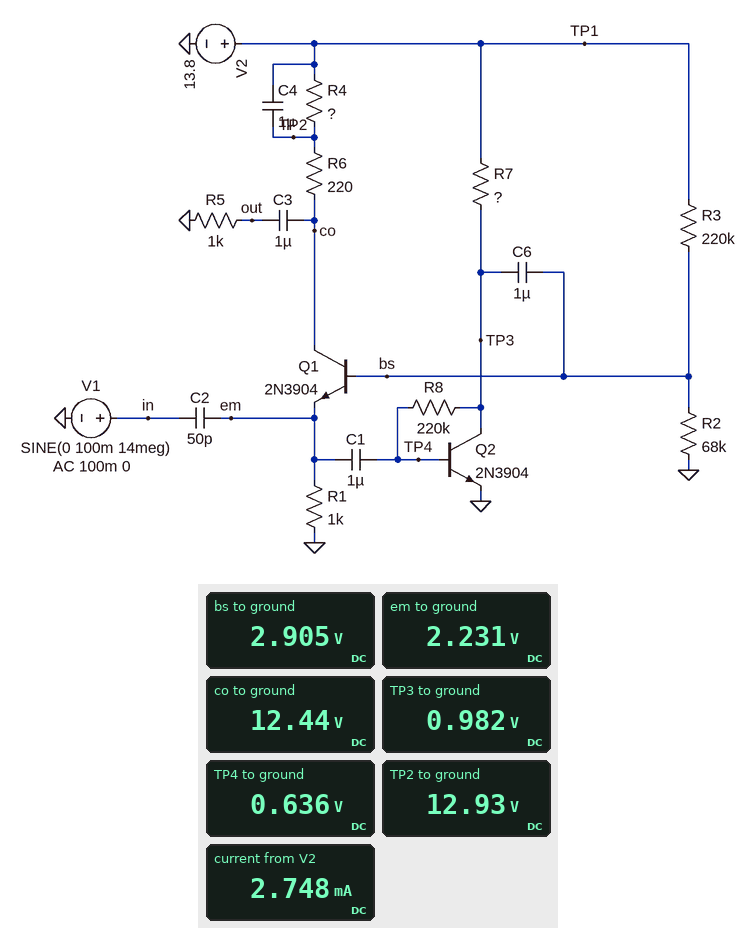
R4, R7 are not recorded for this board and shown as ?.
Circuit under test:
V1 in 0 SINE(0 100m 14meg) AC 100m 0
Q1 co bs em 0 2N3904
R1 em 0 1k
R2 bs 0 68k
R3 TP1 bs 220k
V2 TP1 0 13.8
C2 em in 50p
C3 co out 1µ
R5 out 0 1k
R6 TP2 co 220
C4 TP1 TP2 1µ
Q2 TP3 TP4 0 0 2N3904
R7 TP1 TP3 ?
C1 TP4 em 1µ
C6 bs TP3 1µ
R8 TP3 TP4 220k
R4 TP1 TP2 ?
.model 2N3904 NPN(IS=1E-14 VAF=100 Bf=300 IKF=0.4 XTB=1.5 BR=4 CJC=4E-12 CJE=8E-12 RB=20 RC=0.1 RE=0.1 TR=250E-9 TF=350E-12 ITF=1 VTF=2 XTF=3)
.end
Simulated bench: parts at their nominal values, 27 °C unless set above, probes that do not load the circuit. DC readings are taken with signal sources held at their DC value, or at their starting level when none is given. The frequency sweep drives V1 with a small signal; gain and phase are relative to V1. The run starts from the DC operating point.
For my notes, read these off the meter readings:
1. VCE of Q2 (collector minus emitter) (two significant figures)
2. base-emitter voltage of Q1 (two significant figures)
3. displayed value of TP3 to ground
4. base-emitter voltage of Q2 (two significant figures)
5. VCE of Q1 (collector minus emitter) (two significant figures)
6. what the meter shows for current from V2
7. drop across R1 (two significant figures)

980 mV
670 mV
0.982 V
640 mV
10 V
2.748 mA
2.2 V
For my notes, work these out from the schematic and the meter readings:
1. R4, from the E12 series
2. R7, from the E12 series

390 Ω
27 kΩ
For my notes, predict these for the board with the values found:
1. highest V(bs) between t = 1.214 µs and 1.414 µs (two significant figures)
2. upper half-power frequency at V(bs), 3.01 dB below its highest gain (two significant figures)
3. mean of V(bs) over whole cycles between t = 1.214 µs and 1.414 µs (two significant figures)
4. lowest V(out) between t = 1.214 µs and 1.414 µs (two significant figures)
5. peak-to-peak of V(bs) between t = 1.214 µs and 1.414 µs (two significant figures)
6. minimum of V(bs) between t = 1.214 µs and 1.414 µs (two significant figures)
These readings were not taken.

2.9 V
100 MHz
2.9 V
-81 mV
11 mV
2.9 V
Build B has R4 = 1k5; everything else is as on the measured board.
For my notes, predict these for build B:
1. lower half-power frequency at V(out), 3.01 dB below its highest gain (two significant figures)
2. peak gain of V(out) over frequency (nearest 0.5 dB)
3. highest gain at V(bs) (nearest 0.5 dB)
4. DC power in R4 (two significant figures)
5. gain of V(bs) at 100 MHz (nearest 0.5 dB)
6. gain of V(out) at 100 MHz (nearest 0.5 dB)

74 MHz
24.5 dB
7.5 dB
7.4 mW
4.5 dB
20.0 dB
